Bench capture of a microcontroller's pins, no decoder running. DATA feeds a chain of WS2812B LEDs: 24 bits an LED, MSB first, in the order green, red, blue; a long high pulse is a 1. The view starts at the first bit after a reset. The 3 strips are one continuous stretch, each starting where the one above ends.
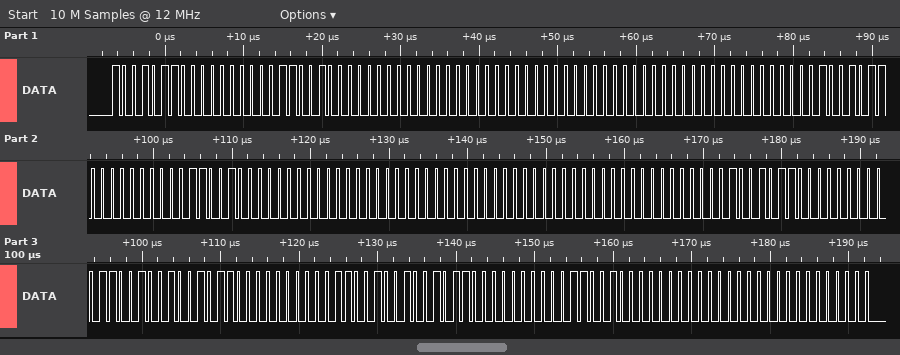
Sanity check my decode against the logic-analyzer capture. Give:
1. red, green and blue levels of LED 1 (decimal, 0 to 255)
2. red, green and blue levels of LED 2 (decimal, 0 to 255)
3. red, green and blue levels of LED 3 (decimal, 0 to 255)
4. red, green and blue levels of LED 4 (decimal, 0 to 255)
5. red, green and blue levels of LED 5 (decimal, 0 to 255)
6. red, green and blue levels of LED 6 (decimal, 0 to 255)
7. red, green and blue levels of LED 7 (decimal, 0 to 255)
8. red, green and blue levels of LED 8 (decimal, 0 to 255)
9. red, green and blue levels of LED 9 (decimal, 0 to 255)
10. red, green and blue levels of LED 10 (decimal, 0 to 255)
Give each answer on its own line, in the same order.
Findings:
0, 150, 100
0, 0, 0
0, 0, 0
0, 150, 100
0, 0, 0
0, 0, 0
0, 150, 100
0, 150, 100
0, 150, 100
0, 0, 0
